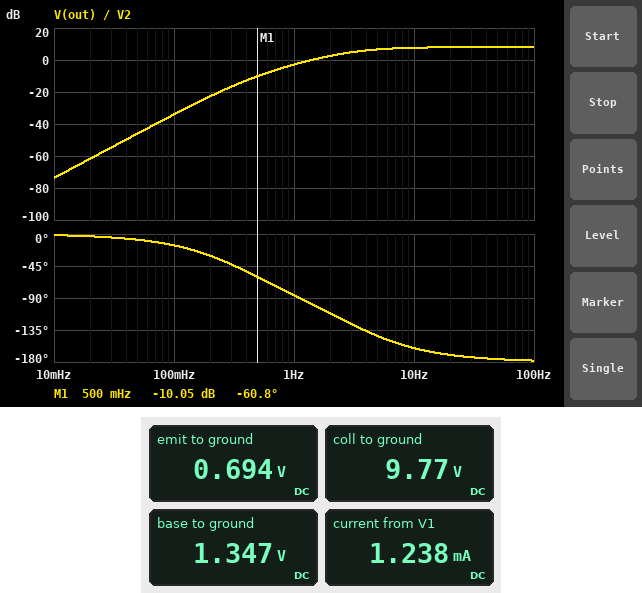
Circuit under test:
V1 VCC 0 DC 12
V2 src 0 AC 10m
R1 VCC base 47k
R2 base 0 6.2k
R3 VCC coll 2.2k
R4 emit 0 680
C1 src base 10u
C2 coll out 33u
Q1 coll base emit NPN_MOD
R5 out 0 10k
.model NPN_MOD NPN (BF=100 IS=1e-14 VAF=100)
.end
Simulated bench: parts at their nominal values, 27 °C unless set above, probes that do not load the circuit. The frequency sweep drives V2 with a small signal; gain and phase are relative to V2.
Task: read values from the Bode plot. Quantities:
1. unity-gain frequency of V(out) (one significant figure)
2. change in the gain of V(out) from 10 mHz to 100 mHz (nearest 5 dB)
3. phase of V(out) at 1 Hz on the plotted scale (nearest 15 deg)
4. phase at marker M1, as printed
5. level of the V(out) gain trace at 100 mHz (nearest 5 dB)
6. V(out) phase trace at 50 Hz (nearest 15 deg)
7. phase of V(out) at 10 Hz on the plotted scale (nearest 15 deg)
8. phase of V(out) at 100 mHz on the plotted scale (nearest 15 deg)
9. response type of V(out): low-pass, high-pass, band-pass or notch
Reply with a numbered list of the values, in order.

1. 1 Hz
2. 40 dB
3. -90 deg
4. -60.8 deg
5. -35 dB
6. -180 deg
7. -165 deg
8. -15 deg
9. high-pass
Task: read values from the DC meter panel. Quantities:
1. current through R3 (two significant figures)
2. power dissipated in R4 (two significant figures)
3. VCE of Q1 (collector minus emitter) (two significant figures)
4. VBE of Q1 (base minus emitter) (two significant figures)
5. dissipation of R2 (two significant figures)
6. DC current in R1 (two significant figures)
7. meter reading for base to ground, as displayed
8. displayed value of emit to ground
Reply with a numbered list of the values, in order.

1. 1.0 mA
2. 710 µW
3. 9.1 V
4. 650 mV
5. 290 µW
6. 230 µA
7. 1.347 V
8. 0.694 V
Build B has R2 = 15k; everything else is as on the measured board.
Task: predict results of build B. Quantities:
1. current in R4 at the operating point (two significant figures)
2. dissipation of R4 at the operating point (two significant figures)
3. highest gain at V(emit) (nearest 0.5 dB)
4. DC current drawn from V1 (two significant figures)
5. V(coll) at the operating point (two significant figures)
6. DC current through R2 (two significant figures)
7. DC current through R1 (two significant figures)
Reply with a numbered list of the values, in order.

1. 2.8 mA
2. 5.4 mW
3. 0 dB
4. 3.0 mA
5. 5.9 V
6. 170 µA
7. 200 µA
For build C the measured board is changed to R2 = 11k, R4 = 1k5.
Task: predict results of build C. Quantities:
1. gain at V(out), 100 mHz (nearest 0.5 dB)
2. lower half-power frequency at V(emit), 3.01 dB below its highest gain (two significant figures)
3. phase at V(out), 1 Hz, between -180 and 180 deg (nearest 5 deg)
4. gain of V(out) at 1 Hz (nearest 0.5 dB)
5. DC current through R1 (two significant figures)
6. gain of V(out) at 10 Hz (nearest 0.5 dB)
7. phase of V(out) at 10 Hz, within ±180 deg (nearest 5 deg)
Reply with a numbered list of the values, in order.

1. -36.5 dB
2. 1.9 Hz
3. -95 deg
4. -6.0 dB
5. 210 µA
6. 1.0 dB
7. -165 deg
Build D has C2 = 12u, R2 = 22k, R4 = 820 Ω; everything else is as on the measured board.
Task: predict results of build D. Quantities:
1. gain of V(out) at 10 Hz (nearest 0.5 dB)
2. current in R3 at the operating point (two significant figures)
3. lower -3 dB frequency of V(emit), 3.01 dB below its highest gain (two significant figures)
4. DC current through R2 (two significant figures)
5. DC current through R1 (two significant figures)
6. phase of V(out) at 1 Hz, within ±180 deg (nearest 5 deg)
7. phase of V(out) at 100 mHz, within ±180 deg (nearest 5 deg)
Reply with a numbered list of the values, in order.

1. 6.5 dB
2. 3.2 mA
3. 1.3 Hz
4. 150 µA
5. 180 µA
6. -80 deg
7. -10 deg
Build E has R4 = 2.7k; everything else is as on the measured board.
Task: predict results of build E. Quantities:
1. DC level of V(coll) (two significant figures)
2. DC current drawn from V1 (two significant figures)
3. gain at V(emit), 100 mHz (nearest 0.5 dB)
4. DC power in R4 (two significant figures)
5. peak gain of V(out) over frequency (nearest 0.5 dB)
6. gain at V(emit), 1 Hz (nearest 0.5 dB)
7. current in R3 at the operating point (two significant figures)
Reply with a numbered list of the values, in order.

1. 11 V
2. 510 µA
3. -29.5 dB
4. 220 µW
5. -4.0 dB
6. -10.0 dB
7. 280 µA
